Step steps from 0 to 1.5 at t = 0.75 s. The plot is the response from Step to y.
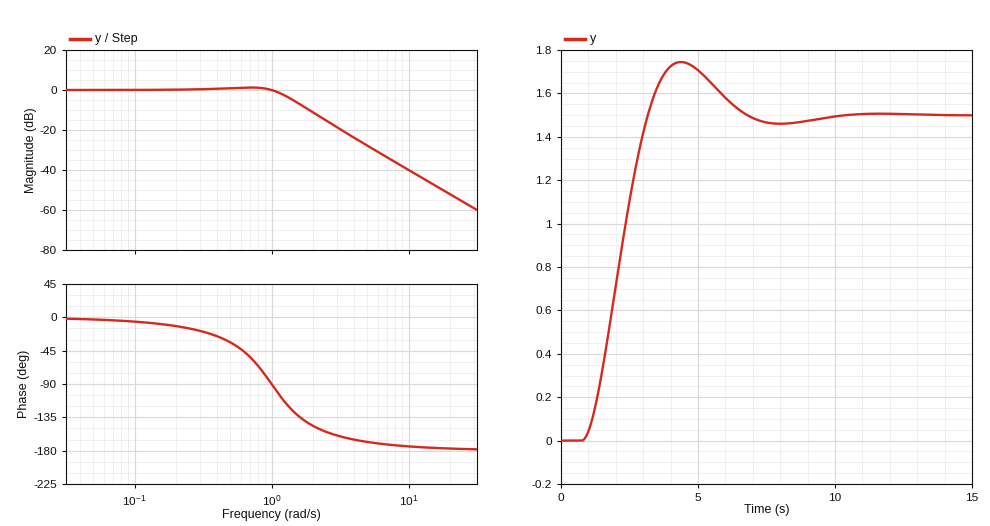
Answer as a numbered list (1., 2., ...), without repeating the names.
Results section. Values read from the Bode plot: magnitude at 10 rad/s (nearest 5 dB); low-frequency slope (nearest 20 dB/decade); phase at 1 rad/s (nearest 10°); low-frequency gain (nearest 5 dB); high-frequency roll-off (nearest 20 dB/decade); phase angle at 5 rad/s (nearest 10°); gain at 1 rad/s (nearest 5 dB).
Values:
1. -40 dB
2. 0 dB/decade
3. -90°
4. 0 dB
5. -40 dB/decade
6. -170°
7. 0 dB
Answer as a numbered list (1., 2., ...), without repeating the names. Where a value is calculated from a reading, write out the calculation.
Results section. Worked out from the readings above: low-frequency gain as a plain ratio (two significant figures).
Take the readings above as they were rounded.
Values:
1. 10^(0 / 20) = 1.0
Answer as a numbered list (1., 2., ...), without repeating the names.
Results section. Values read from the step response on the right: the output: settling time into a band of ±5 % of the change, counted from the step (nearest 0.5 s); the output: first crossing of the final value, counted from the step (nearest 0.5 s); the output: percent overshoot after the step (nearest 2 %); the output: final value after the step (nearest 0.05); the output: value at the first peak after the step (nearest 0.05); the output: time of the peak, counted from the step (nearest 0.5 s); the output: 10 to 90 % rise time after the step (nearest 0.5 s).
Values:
1. 5.5 s
2. 2.5 s
3. 16 %
4. 1.50
5. 1.75
6. 3.5 s
7. 1.5 s
